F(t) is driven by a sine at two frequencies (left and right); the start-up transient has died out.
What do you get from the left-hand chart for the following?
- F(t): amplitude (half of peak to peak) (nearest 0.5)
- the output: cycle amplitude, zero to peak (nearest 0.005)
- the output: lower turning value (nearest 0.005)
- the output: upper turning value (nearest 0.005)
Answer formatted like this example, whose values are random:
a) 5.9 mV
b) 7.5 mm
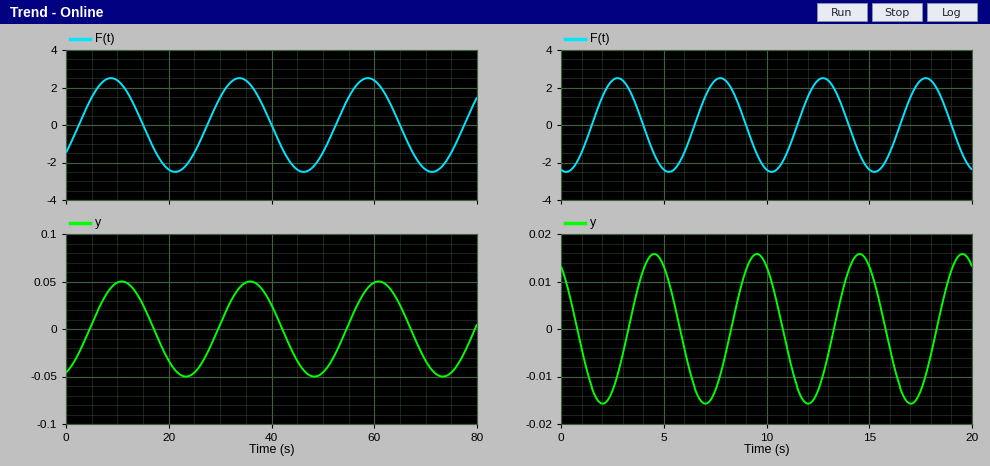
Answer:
a) 2.5
b) 0.050
c) -0.050
d) 0.050
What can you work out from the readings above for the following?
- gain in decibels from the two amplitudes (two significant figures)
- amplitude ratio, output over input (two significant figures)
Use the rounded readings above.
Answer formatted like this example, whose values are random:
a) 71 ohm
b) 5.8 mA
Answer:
a) -34 dB
b) 0.020
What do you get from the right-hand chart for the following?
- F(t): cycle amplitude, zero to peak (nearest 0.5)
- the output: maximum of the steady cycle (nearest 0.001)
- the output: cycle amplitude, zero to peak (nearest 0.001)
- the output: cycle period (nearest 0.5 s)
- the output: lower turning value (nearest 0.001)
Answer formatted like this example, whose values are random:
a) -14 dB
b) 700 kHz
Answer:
a) 2.5
b) 0.016
c) 0.016
d) 5.0 s
e) -0.016
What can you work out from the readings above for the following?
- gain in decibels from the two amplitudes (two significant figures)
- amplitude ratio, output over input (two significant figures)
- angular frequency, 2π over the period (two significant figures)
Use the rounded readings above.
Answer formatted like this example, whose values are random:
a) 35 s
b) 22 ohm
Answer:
a) -44 dB
b) 0.0064
c) 1.3 rad/s
